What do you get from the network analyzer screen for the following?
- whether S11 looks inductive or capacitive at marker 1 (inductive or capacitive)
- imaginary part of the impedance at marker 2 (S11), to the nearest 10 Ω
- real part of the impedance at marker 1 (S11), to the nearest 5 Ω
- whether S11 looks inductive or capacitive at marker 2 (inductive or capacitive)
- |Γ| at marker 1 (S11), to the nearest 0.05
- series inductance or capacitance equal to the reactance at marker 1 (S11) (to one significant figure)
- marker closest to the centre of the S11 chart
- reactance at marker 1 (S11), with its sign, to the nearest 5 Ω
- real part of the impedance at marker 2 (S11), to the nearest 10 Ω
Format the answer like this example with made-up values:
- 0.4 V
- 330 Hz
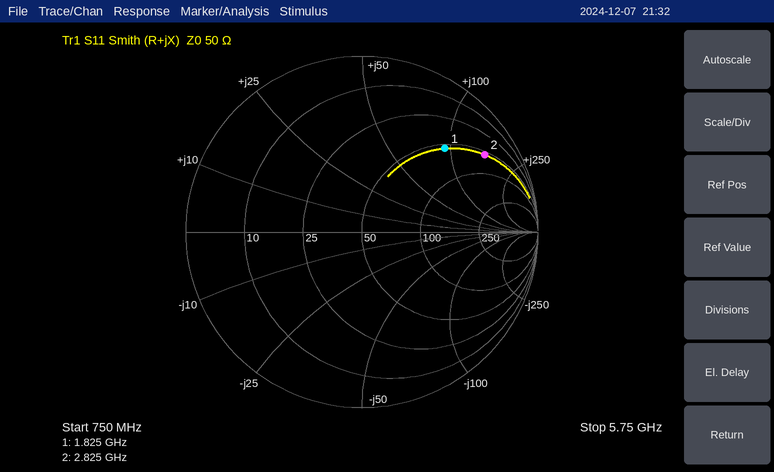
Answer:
- inductive
- +150 Ω
- 55 Ω
- inductive
- 0.65
- 8 nH
- marker 1
- +95 Ω
- 60 Ω
